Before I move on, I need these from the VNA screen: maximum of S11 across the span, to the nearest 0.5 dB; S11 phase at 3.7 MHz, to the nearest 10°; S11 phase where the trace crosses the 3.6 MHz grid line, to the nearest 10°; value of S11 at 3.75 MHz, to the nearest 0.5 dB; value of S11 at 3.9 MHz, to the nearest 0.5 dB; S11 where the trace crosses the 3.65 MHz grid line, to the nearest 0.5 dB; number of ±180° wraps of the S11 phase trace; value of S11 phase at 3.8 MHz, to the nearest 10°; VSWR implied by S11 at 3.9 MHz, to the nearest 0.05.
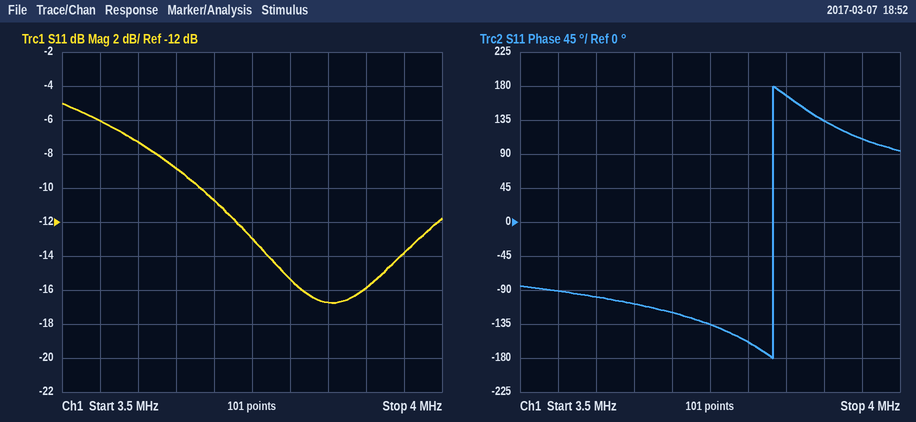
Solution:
-5.0 dB
-120°
-100°
-13.0 dB
-16.0 dB
-9.0 dB
1
-160°
1.40
